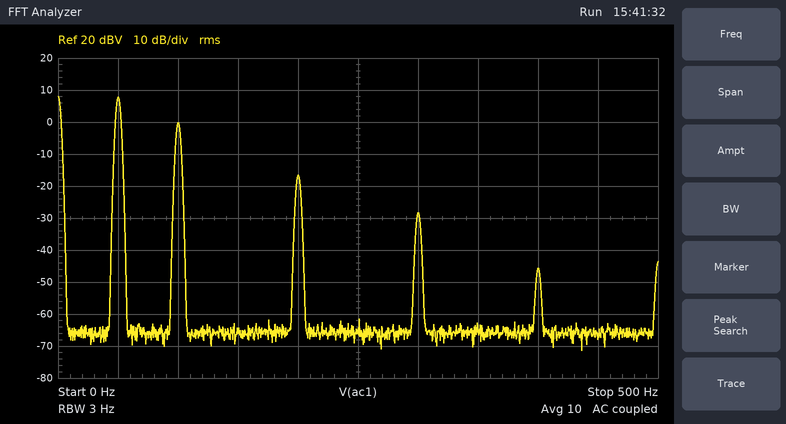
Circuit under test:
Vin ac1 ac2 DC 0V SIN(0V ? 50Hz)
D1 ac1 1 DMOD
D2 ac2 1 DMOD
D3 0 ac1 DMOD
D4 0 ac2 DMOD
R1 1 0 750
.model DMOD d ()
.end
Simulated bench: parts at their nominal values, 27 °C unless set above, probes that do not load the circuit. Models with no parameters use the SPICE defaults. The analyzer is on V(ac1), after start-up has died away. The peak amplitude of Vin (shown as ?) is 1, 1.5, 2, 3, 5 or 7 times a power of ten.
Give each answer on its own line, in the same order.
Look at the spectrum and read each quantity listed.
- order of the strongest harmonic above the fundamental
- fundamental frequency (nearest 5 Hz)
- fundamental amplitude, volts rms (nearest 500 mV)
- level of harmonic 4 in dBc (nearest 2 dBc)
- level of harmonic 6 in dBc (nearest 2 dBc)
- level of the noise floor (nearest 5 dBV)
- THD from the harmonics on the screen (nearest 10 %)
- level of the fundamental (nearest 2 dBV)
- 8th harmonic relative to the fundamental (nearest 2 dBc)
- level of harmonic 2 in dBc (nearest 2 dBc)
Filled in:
2
50 Hz
2.5 V
-24 dBc
-36 dBc
-65 dBV
40 %
8 dBV
-54 dBc
-8 dBc
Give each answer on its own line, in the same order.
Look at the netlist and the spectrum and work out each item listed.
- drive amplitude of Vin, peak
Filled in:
7 V
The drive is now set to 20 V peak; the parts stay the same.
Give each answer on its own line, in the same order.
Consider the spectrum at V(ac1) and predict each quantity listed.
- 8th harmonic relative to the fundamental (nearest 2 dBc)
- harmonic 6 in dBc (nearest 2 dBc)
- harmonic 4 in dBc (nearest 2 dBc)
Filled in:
-36 dBc
-30 dBc
-22 dBc
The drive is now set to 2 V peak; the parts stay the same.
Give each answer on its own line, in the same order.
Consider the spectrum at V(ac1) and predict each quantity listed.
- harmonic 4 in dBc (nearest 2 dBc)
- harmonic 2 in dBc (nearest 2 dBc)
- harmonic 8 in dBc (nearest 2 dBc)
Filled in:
-28 dBc
-14 dBc
-48 dBc
